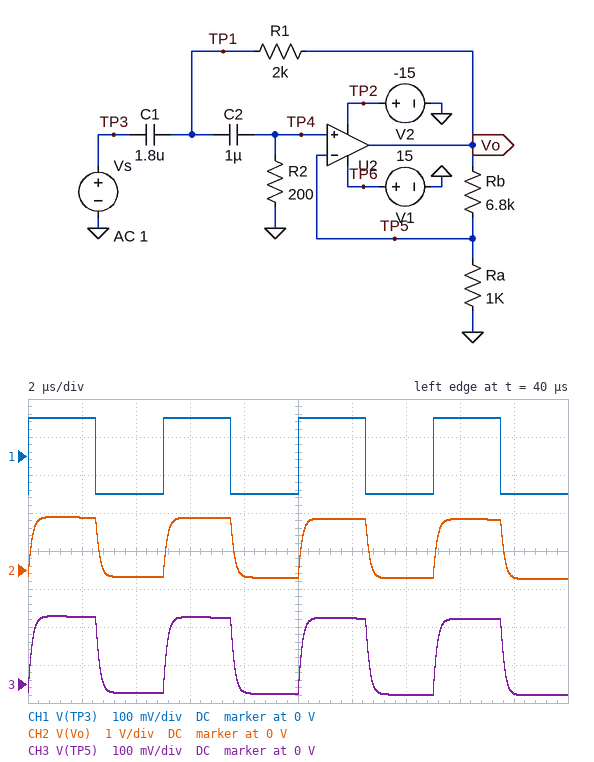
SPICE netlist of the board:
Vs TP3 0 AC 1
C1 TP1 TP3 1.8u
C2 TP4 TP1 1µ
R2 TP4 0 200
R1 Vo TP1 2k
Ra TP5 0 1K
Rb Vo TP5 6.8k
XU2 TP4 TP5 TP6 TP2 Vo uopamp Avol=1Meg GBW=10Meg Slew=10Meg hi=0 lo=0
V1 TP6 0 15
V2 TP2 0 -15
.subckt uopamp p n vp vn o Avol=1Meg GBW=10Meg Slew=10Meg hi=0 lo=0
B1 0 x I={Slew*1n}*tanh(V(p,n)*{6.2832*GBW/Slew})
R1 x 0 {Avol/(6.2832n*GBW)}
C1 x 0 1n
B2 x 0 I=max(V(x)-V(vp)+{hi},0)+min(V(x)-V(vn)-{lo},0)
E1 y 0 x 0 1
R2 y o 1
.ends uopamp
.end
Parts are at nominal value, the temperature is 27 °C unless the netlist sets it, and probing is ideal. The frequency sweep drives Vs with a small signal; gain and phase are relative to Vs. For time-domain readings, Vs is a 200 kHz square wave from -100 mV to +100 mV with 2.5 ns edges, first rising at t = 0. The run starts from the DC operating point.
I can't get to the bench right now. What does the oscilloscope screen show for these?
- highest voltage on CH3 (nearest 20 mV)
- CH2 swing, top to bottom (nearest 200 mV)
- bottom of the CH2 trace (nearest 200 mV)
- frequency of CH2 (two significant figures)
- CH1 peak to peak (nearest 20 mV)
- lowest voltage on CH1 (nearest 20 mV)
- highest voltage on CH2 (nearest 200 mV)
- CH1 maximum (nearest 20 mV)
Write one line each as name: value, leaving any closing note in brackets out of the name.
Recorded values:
highest voltage on CH3: 180 mV
CH2 swing, top to bottom: 1.6 V
bottom of the CH2 trace: -200 mV
frequency of CH2: 200 kHz
CH1 peak to peak: 200 mV
lowest voltage on CH1: -100 mV
highest voltage on CH2: 1.4 V
CH1 maximum: 100 mV
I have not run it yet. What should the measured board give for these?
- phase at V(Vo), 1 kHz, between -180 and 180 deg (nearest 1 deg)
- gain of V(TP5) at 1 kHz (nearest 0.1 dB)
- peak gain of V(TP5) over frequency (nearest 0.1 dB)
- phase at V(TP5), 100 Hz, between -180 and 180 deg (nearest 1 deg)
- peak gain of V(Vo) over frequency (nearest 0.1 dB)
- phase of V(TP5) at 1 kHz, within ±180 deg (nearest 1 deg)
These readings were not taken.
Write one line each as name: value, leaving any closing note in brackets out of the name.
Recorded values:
phase at V(Vo), 1 kHz, between -180 and 180 deg: 44 deg
gain of V(TP5) at 1 kHz: -2.6 dB
peak gain of V(TP5) over frequency: 0 dB
phase at V(TP5), 100 Hz, between -180 and 180 deg: 105 deg
peak gain of V(Vo) over frequency: 17.8 dB
phase of V(TP5) at 1 kHz, within ±180 deg: 44 deg
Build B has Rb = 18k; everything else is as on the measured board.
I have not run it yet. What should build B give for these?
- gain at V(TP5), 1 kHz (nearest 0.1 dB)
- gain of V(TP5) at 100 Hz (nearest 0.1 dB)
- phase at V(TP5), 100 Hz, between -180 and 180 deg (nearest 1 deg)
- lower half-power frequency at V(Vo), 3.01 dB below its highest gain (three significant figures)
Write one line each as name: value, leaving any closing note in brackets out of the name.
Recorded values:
gain at V(TP5), 1 kHz: -0.5 dB
gain of V(TP5) at 100 Hz: -14.1 dB
phase at V(TP5), 100 Hz, between -180 and 180 deg: 120 deg
lower half-power frequency at V(Vo), 3.01 dB below its highest gain: 365 Hz
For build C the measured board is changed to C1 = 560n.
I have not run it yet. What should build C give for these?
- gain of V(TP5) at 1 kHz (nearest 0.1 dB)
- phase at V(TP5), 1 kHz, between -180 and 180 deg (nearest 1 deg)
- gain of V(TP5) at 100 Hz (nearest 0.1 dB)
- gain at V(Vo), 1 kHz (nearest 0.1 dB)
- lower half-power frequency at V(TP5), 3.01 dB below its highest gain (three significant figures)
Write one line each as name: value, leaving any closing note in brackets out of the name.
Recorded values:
gain of V(TP5) at 1 kHz: -3.7 dB
phase at V(TP5), 1 kHz, between -180 and 180 deg: 55 deg
gain of V(TP5) at 100 Hz: -24.2 dB
gain at V(Vo), 1 kHz: 14.1 dB
lower half-power frequency at V(TP5), 3.01 dB below its highest gain: 1.16 kHz
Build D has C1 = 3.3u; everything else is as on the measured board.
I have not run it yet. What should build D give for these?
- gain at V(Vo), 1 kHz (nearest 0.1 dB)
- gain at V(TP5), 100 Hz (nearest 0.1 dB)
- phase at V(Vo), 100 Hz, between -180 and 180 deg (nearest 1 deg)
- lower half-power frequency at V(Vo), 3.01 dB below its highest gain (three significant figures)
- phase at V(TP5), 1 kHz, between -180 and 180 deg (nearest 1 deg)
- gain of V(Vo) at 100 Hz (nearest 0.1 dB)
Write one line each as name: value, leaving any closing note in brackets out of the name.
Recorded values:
gain at V(Vo), 1 kHz: 15.5 dB
gain at V(TP5), 100 Hz: -18.9 dB
phase at V(Vo), 100 Hz, between -180 and 180 deg: 96 deg
lower half-power frequency at V(Vo), 3.01 dB below its highest gain: 850 Hz
phase at V(TP5), 1 kHz, between -180 and 180 deg: 42 deg
gain of V(Vo) at 100 Hz: -1.0 dB
